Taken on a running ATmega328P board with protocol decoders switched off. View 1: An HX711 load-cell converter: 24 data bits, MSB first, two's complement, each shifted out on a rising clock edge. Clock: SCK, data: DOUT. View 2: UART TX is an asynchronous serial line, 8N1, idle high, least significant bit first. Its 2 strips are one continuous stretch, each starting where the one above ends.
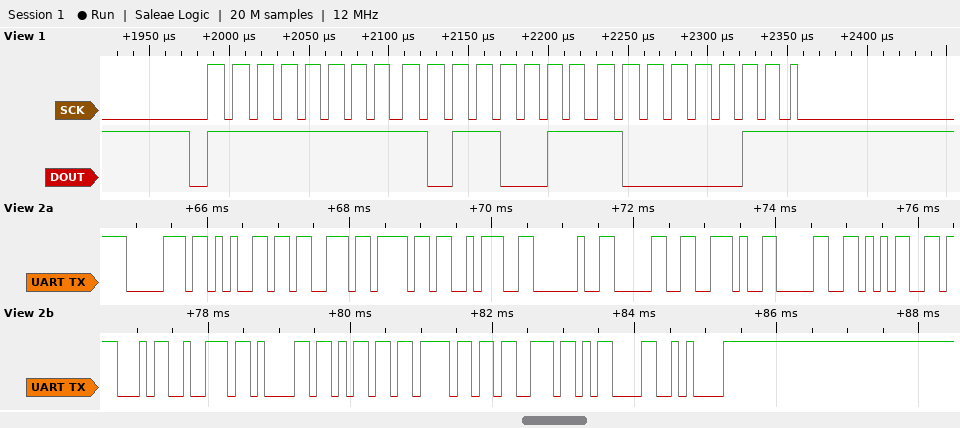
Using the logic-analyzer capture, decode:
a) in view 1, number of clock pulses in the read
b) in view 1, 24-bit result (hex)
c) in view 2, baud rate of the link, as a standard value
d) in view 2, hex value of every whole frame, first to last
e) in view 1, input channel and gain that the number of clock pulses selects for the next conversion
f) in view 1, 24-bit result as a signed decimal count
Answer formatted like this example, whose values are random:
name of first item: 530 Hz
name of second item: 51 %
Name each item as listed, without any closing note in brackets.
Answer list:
in view 1, number of clock pulses in the read: 25
in view 1, 24-bit result: 0xFFB383
in view 2, baud rate of the link, as a standard value: 9600 baud
in view 2, hex value of every whole frame, first to last: 0x70 0x65 0x73 0x6F 0x3A 0x20 0x30 0x2E 0x30 0x35 0x47 0x72 0x61 0x6D 0x6F 0x73 0x0D 0x0A
in view 1, input channel and gain that the number of clock pulses selects for the next conversion: channel A, gain 128
in view 1, 24-bit result as a signed decimal count: -19581
